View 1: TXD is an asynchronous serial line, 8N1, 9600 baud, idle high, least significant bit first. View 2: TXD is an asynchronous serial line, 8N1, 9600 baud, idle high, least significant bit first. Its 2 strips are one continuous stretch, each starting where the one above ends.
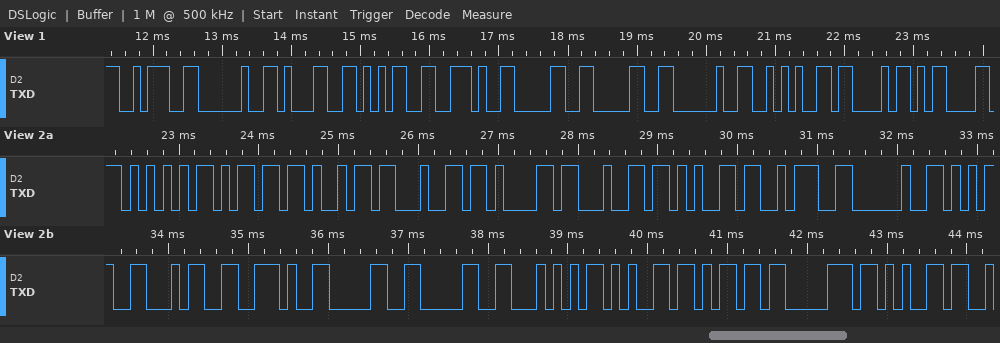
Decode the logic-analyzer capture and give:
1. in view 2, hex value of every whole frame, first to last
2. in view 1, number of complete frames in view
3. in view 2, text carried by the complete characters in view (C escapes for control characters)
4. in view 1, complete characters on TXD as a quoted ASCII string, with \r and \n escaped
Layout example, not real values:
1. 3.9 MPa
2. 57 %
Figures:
1. 55 6D 69 64 61 64 65 3A 20 35 34 2E 30 30 54 65 6D 70 65
2. 11
3. "Umidade: 54.00Tempe"
4. ": 15.00 *C\r"
